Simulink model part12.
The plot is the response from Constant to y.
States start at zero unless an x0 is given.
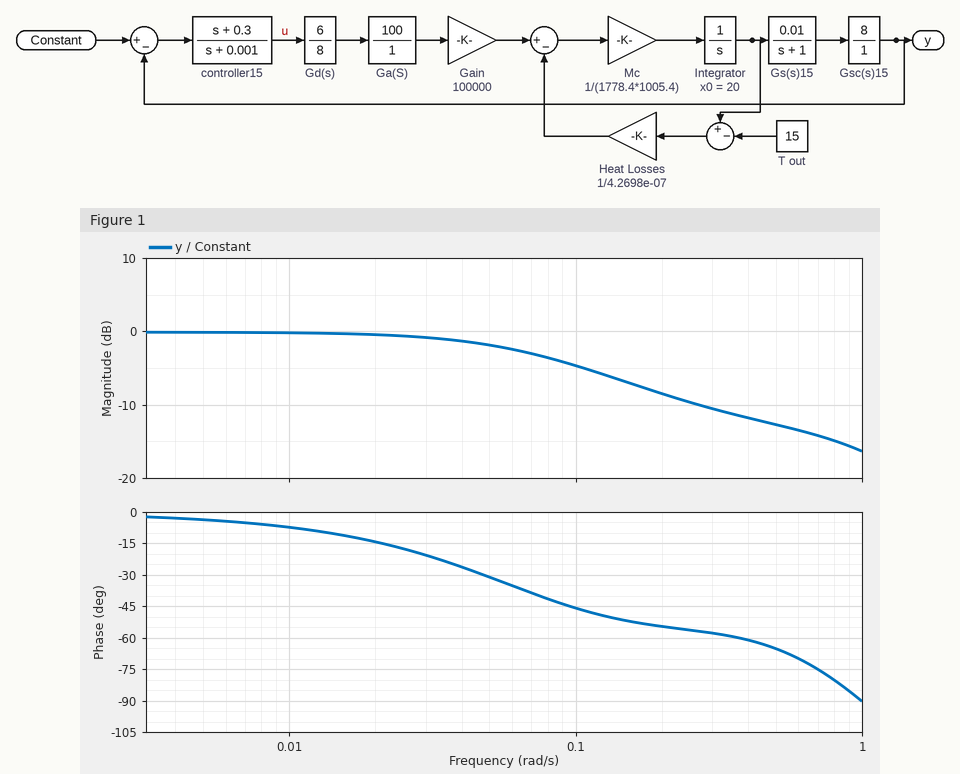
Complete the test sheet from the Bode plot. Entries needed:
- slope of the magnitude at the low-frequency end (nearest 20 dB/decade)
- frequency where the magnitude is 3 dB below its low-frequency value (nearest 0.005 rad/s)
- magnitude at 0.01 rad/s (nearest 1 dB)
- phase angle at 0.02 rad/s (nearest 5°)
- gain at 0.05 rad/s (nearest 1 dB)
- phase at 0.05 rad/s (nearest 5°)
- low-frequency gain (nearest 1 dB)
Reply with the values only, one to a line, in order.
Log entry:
0 dB/decade
0.070 rad/s
0 dB
-15°
-2 dB
-30°
0 dB
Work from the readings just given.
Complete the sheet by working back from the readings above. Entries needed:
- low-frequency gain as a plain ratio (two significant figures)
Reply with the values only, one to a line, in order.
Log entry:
1.0
